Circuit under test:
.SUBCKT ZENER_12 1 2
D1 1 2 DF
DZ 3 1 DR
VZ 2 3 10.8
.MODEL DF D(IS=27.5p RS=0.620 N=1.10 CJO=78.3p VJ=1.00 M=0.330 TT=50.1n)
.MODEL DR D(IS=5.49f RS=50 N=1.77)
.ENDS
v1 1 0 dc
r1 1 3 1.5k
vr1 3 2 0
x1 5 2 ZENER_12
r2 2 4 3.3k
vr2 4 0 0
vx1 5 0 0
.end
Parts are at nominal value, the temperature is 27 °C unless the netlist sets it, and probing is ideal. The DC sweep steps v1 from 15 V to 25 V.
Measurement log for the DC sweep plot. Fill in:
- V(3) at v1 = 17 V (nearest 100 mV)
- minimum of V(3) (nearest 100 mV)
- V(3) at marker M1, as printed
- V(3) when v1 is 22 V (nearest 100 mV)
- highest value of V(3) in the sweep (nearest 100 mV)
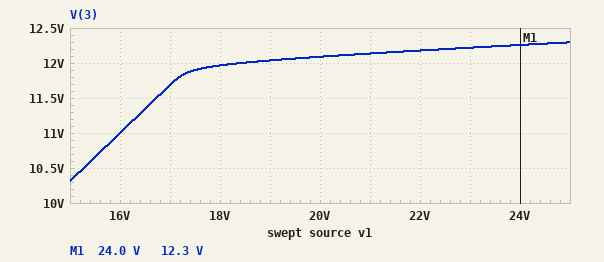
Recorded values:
11.7 V
10.3 V
12.3 V
12.2 V
12.3 V
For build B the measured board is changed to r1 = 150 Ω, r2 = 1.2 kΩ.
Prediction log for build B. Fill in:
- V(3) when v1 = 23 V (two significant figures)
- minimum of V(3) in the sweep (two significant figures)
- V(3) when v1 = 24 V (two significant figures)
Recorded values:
14 V
12 V
15 V
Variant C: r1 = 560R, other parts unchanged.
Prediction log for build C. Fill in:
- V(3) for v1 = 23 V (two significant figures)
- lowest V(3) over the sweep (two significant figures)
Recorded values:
13 V
12 V
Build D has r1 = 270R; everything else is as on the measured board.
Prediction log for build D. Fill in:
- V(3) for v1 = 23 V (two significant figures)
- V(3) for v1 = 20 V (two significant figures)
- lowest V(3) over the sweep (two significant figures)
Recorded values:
14 V
13 V
12 V
